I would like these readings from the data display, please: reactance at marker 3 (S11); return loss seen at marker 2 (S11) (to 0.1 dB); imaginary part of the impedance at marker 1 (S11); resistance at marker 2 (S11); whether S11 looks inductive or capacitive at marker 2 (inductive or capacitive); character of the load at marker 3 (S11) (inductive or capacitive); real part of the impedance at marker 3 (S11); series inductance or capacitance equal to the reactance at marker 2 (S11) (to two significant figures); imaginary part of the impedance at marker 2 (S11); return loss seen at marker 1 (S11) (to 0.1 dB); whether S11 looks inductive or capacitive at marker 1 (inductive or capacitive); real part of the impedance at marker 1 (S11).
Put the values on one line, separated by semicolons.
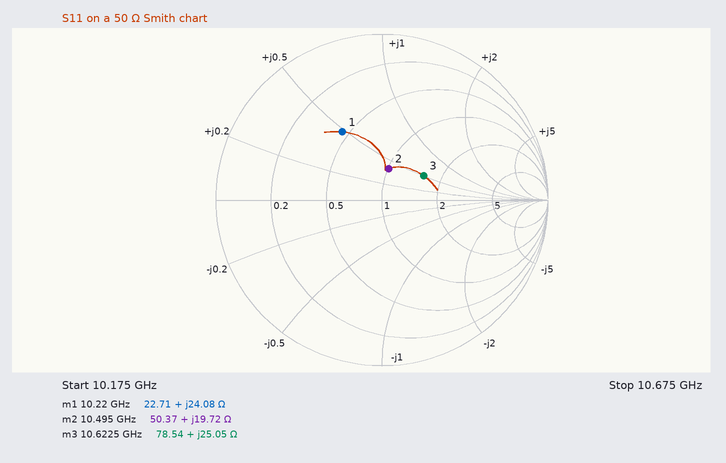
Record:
+25.05 Ω; 14.3 dB; +24.08 Ω; 50.37 Ω; inductive; inductive; 78.54 Ω; 300 pH; +19.72 Ω; 6.5 dB; inductive; 22.71 Ω
